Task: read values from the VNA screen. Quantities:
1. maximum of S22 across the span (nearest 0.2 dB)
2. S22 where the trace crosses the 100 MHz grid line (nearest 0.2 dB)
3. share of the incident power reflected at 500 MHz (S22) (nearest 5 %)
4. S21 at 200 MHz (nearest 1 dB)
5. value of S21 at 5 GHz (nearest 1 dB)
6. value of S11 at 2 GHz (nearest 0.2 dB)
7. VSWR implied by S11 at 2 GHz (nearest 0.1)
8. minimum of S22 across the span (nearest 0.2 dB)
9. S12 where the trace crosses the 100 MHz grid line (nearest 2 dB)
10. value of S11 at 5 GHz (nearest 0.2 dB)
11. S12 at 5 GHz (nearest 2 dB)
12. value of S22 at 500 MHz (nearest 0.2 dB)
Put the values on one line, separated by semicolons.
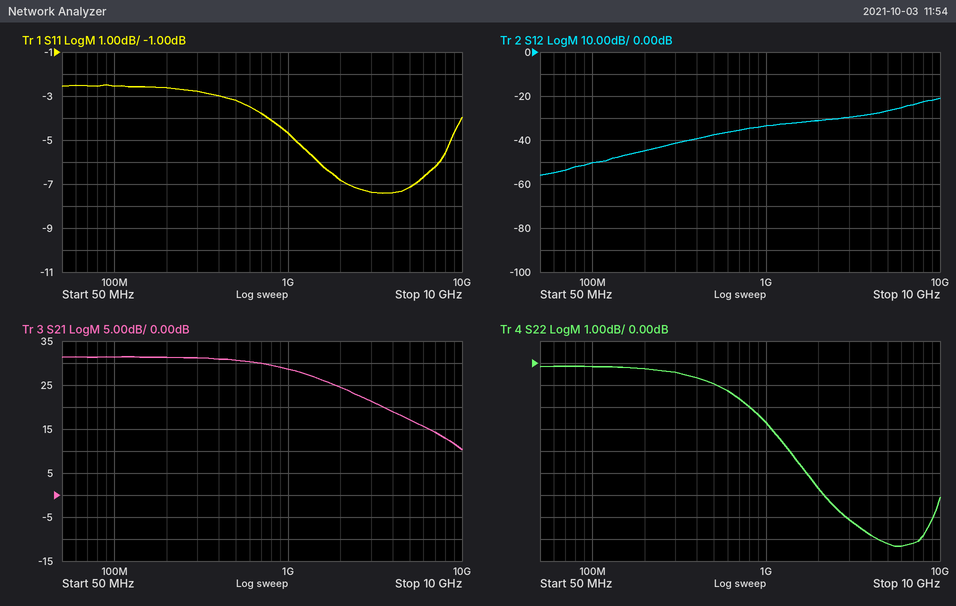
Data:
-0.2 dB; -0.2 dB; 80 %; 31 dB; 17 dB; -6.8 dB; 2.7; -8.4 dB; -50 dB; -7.2 dB; -26 dB; -1.0 dB
